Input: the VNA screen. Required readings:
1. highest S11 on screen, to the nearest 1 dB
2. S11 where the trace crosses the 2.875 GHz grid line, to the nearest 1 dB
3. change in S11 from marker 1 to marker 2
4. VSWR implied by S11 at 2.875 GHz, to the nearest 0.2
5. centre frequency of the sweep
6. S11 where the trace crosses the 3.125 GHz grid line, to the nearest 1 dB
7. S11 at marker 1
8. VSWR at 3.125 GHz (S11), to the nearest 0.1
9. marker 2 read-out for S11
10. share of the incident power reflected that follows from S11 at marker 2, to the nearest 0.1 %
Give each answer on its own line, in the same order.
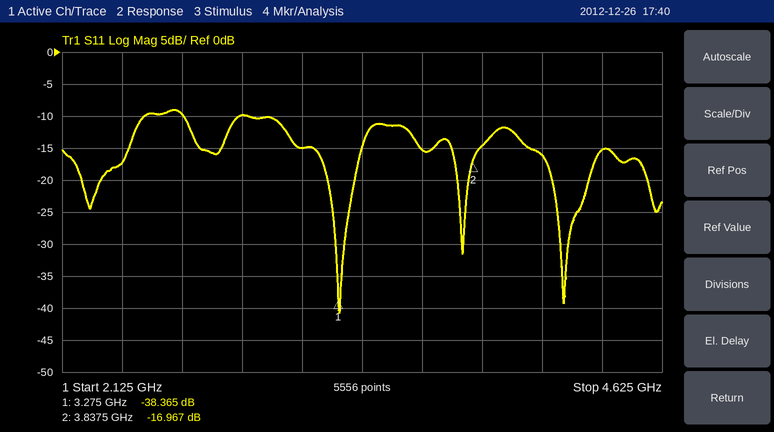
-9 dB
-10 dB
21.398 dB
2.0
3.375 GHz
-15 dB
-38.365 dB
1.4
-16.967 dB
2.0 %
